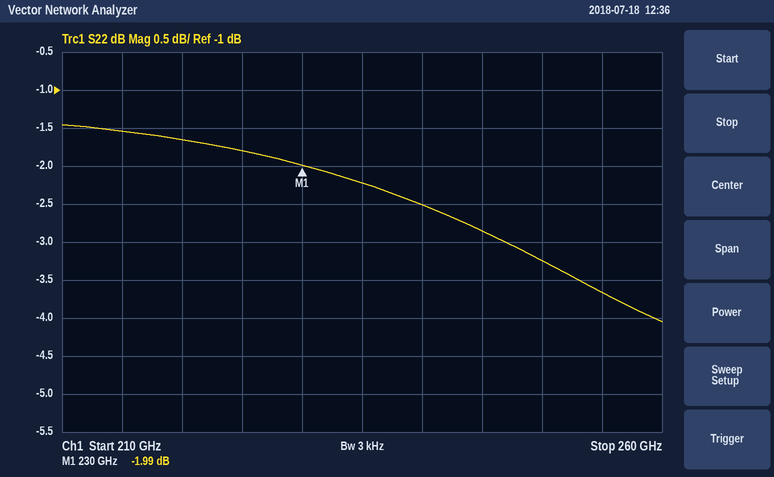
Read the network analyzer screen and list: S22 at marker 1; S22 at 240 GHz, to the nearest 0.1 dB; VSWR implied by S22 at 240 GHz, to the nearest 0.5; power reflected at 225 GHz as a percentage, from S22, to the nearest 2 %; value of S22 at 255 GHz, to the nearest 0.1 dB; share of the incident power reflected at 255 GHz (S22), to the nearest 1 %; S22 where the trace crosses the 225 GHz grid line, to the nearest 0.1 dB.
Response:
-1.99 dB
-2.5 dB
7.0
66 %
-3.7 dB
43 %
-1.8 dB
